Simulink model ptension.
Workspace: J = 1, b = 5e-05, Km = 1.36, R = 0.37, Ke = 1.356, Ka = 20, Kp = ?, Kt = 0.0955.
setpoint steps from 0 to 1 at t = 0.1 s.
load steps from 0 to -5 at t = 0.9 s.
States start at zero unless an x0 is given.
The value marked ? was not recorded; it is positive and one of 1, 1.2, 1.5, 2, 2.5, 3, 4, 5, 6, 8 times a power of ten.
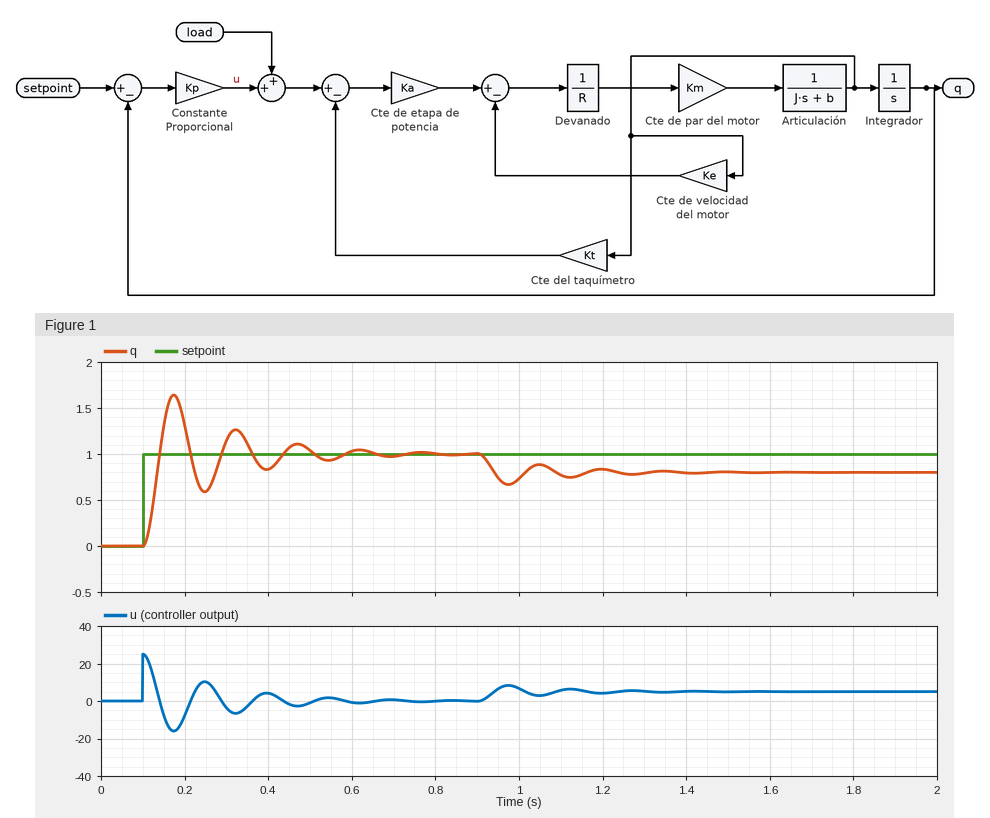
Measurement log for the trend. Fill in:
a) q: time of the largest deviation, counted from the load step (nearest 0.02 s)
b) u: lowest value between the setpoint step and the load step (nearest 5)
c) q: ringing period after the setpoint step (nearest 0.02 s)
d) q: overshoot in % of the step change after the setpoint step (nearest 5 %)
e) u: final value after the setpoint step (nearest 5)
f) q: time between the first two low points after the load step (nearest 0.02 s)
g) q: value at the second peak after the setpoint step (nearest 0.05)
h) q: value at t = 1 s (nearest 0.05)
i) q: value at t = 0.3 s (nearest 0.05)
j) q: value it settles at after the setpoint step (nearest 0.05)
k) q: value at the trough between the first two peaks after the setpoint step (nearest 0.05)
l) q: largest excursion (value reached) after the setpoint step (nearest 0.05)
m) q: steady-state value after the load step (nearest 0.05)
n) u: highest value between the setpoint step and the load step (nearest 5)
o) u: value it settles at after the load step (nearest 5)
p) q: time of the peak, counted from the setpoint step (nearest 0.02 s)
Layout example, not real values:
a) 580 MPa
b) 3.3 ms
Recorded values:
a) 0.08 s
b) -15
c) 0.14 s
d) 65 %
e) 0
f) 0.14 s
g) 1.25
h) 0.75
i) 1.15
j) 1.00
k) 0.60
l) 1.65
m) 0.80
n) 25
o) 5
p) 0.08 s
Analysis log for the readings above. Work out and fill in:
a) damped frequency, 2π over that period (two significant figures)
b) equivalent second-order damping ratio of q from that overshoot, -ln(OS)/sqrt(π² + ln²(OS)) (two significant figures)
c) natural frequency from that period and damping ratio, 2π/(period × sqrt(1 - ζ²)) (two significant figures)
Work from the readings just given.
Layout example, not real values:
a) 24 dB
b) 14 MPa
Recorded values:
a) 45 rad/s
b) 0.14
c) 45 rad/s
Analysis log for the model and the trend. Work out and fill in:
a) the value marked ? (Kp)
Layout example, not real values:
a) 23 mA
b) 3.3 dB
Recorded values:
a) 25
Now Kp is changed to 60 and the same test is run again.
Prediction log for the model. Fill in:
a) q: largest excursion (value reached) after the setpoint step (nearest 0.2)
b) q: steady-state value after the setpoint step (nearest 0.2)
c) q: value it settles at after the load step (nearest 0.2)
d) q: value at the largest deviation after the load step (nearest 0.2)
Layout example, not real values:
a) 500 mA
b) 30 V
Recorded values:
a) 1.8
b) 1.0
c) 1.0
d) 0.8
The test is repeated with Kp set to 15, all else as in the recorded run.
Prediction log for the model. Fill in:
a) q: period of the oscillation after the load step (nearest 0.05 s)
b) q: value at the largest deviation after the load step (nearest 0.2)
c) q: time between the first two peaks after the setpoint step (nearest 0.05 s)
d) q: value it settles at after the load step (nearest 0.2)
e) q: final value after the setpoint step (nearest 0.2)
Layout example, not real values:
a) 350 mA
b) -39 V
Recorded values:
a) 0.20 s
b) 0.4
c) 0.20 s
d) 0.6
e) 1.0
